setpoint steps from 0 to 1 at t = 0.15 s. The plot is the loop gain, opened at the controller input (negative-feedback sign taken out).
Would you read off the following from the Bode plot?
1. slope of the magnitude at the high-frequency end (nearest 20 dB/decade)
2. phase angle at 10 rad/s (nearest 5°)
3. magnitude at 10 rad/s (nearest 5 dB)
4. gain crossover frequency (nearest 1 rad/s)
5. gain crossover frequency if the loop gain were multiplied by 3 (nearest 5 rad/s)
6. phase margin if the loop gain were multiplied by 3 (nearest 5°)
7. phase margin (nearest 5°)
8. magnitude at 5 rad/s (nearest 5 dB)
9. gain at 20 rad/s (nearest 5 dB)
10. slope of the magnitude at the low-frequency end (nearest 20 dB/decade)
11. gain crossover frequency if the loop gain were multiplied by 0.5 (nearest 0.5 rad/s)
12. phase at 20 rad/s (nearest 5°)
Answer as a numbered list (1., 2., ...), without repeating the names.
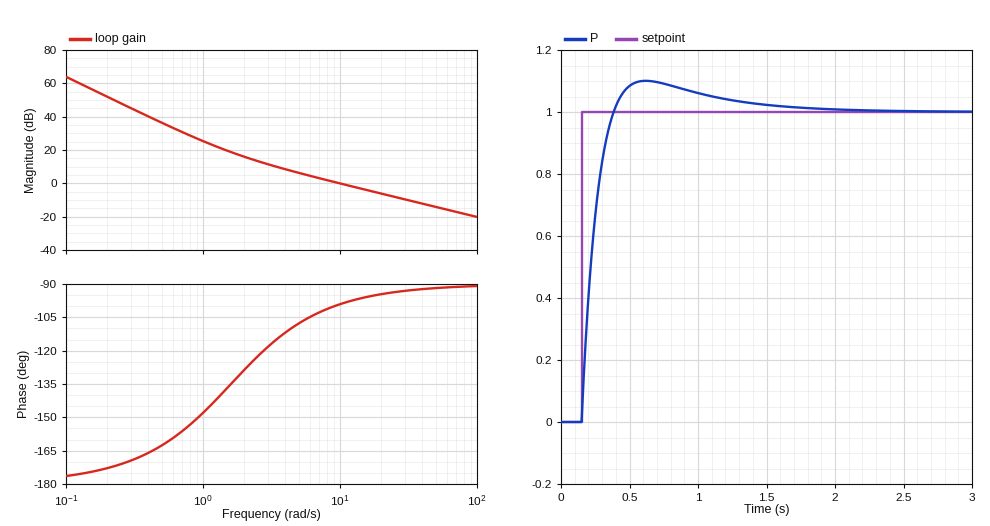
1. -20 dB/decade
2. -100°
3. 0 dB
4. 10 rad/s
5. 30 rad/s
6. 85°
7. 80°
8. 5 dB
9. -5 dB
10. -40 dB/decade
11. 5.0 rad/s
12. -95°
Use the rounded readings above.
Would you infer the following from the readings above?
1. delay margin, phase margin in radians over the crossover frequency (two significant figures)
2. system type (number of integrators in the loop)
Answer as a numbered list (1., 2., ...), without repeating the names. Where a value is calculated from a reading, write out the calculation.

1. 80 × π / 180 / 10 = 0.14 s
2. 2
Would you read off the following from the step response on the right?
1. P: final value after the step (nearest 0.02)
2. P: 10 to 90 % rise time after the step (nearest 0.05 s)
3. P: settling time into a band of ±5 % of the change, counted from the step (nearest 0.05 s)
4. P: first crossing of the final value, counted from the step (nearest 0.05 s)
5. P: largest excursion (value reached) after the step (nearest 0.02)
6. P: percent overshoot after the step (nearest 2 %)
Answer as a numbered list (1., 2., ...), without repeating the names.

1. 1.00
2. 0.15 s
3. 0.95 s
4. 0.25 s
5. 1.10
6. 10 %
